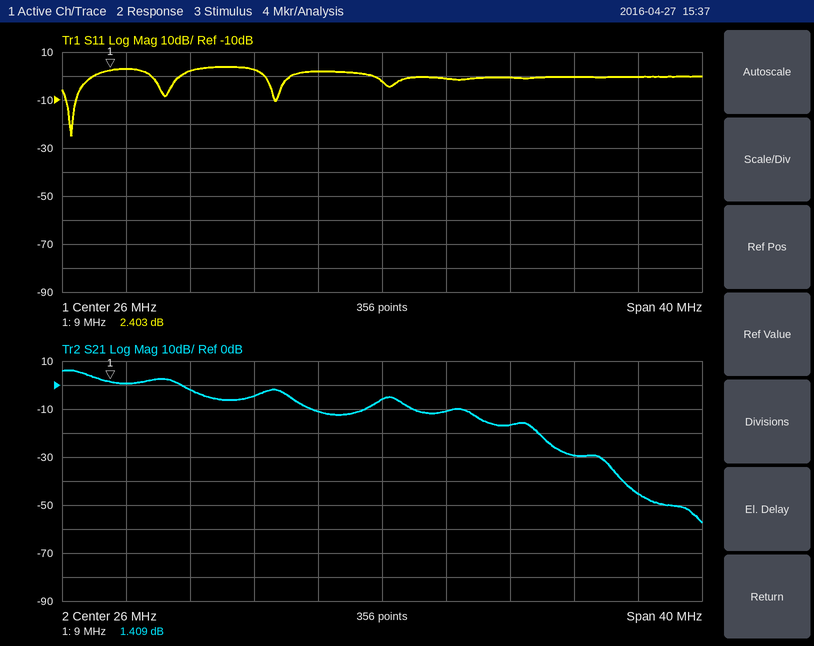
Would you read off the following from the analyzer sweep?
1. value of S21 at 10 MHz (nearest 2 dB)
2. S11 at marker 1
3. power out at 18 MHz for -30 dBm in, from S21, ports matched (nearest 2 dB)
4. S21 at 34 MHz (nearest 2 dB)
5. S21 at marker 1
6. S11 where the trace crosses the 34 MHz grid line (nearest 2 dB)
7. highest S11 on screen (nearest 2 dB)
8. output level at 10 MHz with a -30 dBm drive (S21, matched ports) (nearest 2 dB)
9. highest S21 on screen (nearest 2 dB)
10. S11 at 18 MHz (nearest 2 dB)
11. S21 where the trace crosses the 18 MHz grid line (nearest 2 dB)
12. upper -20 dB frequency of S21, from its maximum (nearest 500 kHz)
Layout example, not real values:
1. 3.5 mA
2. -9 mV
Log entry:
1. 0 dB
2. 2.403 dB
3. -34 dBm
4. -16 dB
5. 1.409 dB
6. 0 dB
7. 4 dB
8. -30 dBm
9. 6 dB
10. 2 dB
11. -4 dB
12. 32.0 MHz
